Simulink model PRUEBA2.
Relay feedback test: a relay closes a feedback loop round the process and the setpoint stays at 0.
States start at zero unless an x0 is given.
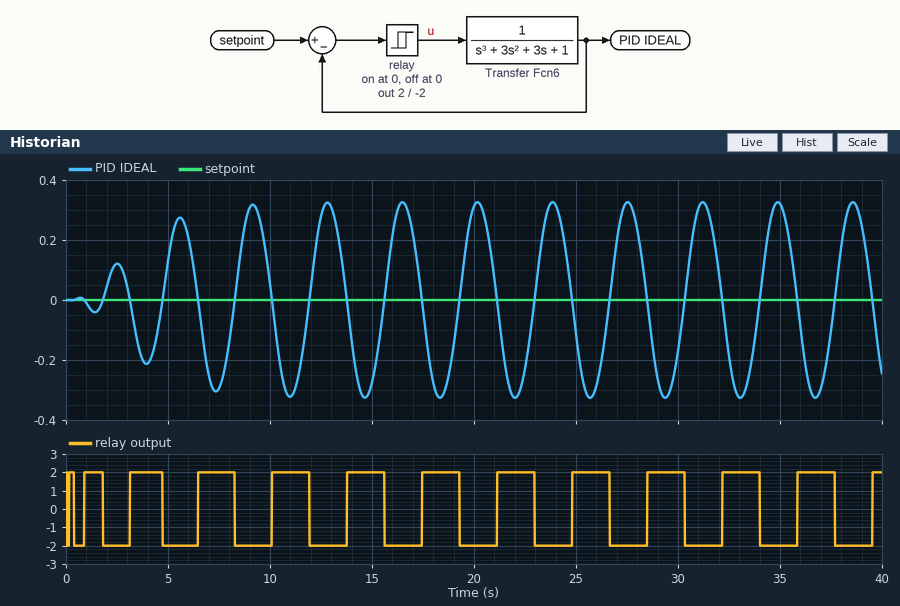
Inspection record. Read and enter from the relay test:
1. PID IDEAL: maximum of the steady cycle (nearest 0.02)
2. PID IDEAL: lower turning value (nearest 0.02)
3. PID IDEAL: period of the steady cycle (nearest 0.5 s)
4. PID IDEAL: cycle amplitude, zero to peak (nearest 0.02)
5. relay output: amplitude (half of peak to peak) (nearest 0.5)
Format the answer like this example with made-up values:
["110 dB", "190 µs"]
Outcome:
["0.32", "-0.32", "3.5 s", "0.32", "2.0"]
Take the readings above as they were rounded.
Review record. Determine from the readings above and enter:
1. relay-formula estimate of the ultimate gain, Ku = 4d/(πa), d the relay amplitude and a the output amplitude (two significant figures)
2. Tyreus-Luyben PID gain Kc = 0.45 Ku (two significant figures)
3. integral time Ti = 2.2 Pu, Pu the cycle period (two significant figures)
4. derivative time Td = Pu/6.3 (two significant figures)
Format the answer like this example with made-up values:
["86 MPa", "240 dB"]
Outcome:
["8.0", "3.6", "7.7 s", "0.56 s"]
